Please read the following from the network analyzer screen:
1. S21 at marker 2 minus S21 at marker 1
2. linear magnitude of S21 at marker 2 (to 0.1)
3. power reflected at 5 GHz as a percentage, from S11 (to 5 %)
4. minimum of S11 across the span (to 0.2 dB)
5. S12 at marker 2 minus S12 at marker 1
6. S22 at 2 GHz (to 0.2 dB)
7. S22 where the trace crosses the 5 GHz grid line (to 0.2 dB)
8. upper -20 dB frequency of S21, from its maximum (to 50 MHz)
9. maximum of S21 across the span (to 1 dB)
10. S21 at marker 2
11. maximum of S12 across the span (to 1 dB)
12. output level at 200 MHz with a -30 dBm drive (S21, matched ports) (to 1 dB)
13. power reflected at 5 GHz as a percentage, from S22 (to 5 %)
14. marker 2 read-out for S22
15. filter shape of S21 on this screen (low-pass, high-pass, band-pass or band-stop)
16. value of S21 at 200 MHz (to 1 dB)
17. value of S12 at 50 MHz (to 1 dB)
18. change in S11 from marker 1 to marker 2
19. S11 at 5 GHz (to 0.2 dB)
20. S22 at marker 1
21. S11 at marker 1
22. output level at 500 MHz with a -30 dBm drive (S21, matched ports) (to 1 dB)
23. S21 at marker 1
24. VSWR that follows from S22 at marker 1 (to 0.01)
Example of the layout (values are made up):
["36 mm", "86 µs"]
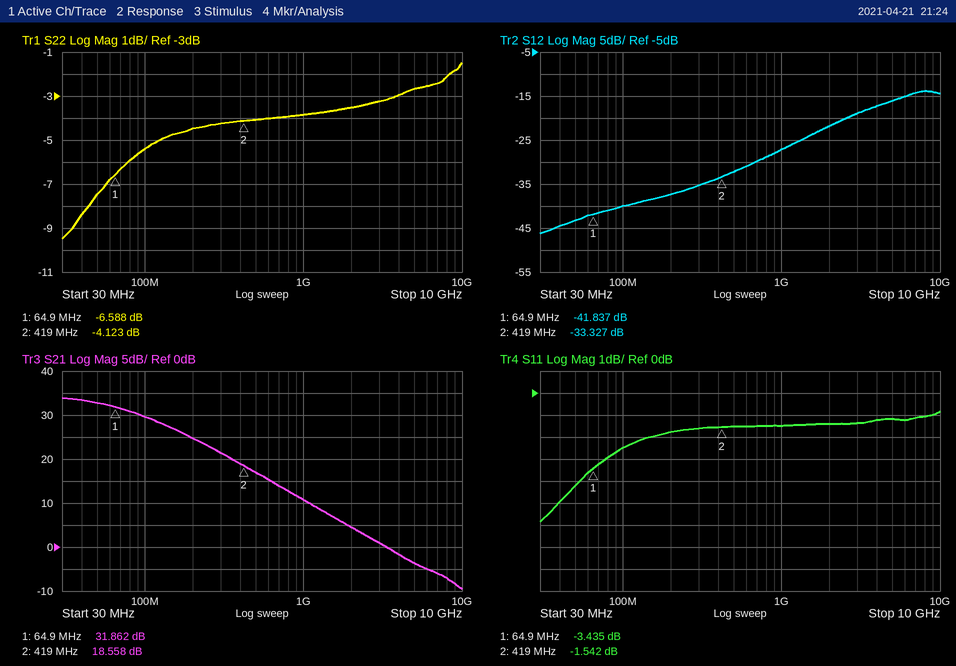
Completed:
["-13.304 dB", "8.5", "75 %", "-5.8 dB", "8.510 dB", "-3.6 dB", "-2.6 dB", "700 MHz", "34 dB", "18.558 dB", "-14 dB", "-5 dBm", "55 %", "-4.123 dB", "low-pass", "25 dB", "-43 dB", "1.893 dB", "-1.2 dB", "-6.588 dB", "-3.435 dB", "-13 dBm", "31.862 dB", "2.76"]
